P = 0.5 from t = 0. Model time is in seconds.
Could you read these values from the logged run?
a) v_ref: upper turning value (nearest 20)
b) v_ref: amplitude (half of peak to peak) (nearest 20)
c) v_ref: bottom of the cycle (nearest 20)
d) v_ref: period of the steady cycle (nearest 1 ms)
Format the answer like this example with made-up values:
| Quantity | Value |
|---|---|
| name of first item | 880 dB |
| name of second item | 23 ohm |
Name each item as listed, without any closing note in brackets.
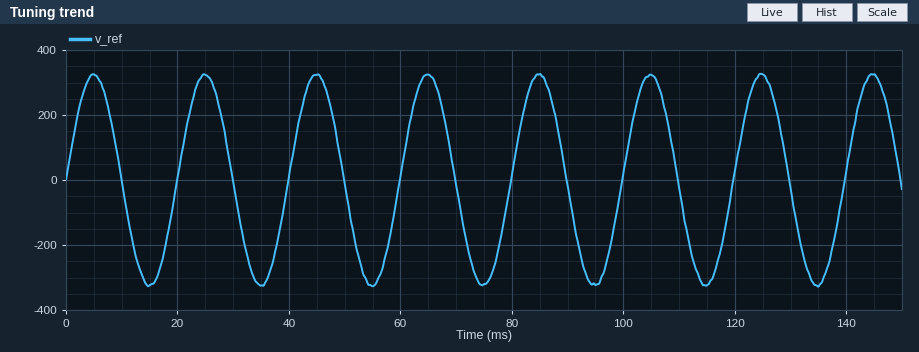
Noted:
| Quantity | Value |
|---|---|
| v_ref: upper turning value | 320 |
| v_ref: amplitude (half of peak to peak) | 320 |
| v_ref: bottom of the cycle | -320 |
| v_ref: period of the steady cycle | 20 ms |
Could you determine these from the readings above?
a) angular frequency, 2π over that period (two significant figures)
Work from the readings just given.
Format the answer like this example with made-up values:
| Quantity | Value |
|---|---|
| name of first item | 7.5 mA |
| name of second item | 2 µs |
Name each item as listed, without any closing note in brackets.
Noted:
| Quantity | Value |
|---|---|
| angular frequency, 2π over that period | 0.31 rad/ms |
